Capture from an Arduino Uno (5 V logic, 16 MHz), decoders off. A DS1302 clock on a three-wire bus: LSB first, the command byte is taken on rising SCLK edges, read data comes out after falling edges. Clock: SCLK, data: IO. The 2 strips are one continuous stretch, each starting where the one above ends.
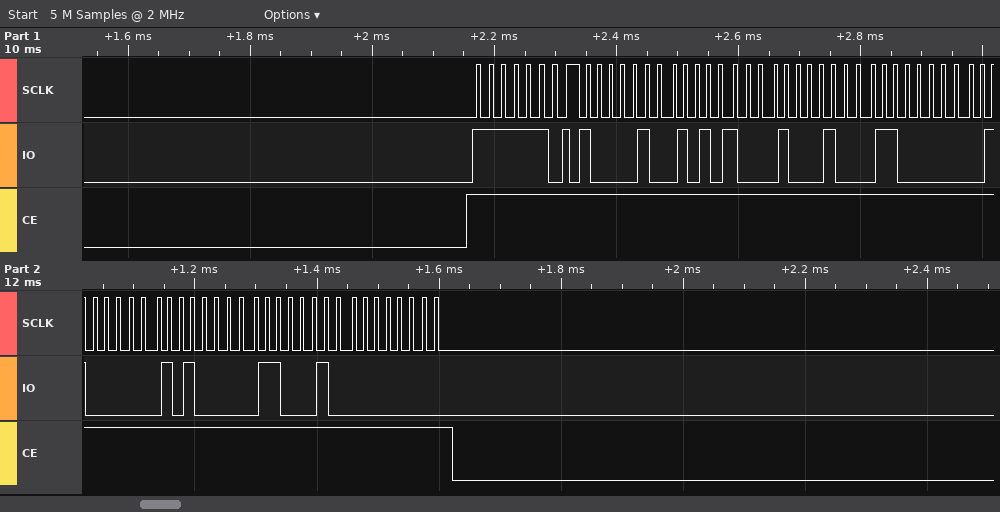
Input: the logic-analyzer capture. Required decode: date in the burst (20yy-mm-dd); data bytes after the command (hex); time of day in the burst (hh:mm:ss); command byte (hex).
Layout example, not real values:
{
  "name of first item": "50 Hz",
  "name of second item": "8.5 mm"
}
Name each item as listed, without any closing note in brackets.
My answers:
{
  "date in the burst": "2023-02-03",
  "data bytes after the command": "21 15 11 03 02 05 23 00",
  "time of day in the burst": "11:15:21",
  "command byte": "0xBF"
}
